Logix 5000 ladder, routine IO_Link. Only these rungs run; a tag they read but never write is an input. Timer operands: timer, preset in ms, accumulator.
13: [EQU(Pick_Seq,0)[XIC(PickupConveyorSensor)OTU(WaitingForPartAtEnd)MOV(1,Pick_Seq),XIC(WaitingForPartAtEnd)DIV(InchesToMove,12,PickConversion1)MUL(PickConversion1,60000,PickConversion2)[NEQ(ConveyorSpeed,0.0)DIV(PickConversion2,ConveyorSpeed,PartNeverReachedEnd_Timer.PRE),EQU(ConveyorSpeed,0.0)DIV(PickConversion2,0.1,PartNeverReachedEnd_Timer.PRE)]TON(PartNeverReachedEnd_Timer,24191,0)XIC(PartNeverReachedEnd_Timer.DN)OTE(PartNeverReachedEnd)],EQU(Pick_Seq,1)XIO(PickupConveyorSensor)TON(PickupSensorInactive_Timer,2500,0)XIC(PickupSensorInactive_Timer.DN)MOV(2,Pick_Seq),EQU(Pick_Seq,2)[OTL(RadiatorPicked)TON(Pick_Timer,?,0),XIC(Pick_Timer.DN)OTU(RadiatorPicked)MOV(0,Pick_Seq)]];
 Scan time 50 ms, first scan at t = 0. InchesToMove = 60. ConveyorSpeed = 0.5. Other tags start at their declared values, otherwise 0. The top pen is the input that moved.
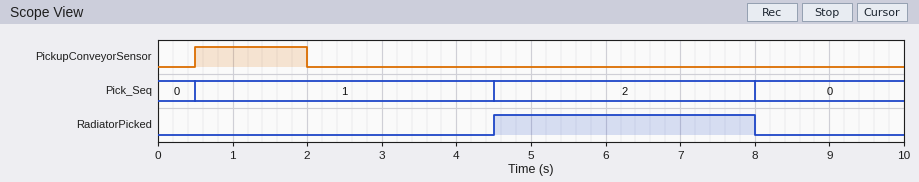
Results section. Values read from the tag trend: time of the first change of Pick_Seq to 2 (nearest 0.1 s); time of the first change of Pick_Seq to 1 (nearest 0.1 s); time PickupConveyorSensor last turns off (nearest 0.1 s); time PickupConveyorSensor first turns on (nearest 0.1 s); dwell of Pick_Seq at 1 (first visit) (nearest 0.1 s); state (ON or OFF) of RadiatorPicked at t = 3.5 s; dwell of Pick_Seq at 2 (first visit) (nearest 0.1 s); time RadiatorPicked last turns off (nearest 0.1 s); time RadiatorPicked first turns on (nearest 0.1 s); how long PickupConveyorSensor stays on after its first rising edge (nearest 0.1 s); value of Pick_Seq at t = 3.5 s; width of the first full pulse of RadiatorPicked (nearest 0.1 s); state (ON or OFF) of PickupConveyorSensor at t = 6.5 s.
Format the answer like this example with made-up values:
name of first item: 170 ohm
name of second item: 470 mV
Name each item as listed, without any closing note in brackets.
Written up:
time of the first change of Pick_Seq to 2: 4.5 s
time of the first change of Pick_Seq to 1: 0.5 s
time PickupConveyorSensor last turns off: 2.0 s
time PickupConveyorSensor first turns on: 0.5 s
dwell of Pick_Seq at 1 (first visit): 4.0 s
state (ON or OFF) of RadiatorPicked at t = 3.5 s: OFF
dwell of Pick_Seq at 2 (first visit): 3.5 s
time RadiatorPicked last turns off: 8.0 s
time RadiatorPicked first turns on: 4.5 s
how long PickupConveyorSensor stays on after its first rising edge: 1.5 s
value of Pick_Seq at t = 3.5 s: 1
width of the first full pulse of RadiatorPicked: 3.5 s
state (ON or OFF) of PickupConveyorSensor at t = 6.5 s: OFF
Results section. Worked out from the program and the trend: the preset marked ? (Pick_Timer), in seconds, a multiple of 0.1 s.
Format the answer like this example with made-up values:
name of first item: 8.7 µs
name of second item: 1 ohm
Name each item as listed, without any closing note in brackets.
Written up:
the preset marked ? (Pick_Timer), in seconds, a multiple of 0.1 s: 3.5 s
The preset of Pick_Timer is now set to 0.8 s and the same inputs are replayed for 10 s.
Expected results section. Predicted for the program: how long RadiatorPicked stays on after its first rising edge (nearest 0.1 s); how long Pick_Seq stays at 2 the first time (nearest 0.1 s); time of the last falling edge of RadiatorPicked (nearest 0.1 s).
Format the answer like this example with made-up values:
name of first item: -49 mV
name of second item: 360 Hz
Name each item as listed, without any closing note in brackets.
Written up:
how long RadiatorPicked stays on after its first rising edge: 0.8 s
how long Pick_Seq stays at 2 the first time: 0.8 s
time of the last falling edge of RadiatorPicked: 5.3 s
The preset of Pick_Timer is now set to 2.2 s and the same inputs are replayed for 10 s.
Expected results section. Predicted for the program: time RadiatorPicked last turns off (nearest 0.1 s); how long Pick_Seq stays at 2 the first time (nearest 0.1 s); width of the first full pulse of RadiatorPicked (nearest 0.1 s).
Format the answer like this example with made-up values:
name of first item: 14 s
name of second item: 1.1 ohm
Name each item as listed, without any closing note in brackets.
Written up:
time RadiatorPicked last turns off: 6.7 s
how long Pick_Seq stays at 2 the first time: 2.2 s
width of the first full pulse of RadiatorPicked: 2.2 s
